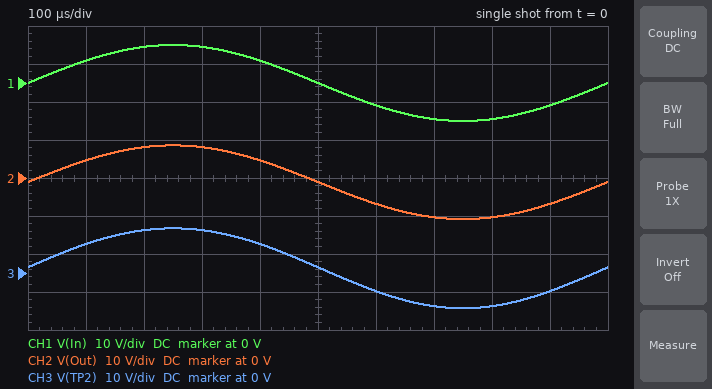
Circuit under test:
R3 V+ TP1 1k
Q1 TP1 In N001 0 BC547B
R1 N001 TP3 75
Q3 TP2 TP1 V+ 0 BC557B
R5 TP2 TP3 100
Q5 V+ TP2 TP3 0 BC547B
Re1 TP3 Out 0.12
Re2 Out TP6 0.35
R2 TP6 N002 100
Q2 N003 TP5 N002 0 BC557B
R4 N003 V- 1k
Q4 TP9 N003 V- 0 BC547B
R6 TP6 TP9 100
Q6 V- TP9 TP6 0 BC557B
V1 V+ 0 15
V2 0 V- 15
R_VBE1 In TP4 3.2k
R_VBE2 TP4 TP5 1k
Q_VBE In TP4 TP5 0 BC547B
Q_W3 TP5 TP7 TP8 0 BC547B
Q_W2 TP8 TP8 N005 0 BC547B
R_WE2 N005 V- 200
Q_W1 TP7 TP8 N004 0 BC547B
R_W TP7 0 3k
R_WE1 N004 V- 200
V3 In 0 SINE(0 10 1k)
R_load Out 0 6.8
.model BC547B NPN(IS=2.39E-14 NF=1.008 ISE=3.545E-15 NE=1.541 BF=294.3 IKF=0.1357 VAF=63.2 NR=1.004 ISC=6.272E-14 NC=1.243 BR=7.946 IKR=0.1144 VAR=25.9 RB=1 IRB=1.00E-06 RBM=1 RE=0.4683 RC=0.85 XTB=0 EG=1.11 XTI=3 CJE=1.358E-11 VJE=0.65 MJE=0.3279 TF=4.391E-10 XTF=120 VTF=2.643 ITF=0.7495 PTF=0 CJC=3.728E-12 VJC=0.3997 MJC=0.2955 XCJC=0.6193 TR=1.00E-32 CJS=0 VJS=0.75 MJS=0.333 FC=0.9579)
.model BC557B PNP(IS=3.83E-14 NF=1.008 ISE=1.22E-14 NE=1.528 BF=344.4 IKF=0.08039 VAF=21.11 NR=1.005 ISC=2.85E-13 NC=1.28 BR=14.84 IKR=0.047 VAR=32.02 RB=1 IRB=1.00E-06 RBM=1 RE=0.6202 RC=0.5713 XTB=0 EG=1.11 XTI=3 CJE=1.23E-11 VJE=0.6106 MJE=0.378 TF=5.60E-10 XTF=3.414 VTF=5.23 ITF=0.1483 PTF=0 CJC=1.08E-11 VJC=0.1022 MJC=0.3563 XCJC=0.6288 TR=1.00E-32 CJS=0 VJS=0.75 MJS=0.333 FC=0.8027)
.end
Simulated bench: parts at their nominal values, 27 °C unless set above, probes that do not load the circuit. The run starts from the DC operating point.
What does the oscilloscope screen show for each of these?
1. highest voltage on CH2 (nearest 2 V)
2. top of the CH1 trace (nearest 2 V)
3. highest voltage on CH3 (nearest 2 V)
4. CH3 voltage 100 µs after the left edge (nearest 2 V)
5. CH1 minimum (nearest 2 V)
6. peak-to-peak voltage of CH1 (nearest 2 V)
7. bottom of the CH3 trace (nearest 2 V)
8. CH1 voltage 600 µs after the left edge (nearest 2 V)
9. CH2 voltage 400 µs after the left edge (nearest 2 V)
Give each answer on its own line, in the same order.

8 V
10 V
12 V
8 V
-10 V
20 V
-10 V
-6 V
4 V
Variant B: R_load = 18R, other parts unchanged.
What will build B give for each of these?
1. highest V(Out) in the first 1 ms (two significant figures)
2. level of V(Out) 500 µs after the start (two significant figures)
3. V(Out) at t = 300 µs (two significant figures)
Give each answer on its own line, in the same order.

8.7 V
-1.1 V
8.3 V
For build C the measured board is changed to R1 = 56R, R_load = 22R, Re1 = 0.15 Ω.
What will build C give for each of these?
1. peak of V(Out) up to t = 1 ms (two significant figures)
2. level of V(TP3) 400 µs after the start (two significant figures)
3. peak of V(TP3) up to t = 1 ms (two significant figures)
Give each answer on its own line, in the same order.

8.7 V
5.1 V
9.2 V
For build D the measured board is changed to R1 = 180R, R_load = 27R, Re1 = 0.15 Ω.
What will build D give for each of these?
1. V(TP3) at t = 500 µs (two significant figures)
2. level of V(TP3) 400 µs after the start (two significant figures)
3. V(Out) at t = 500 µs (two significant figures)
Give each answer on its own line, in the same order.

-870 mV
4.9 V
-1.2 V
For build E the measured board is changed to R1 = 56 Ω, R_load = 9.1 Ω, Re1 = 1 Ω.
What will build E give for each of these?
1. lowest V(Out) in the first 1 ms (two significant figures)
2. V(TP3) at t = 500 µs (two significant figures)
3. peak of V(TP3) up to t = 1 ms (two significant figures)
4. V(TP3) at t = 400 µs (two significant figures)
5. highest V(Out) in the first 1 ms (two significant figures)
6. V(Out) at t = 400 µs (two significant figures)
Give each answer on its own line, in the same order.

-11 V
-670 mV
9.3 V
5.2 V
8.0 V
4.0 V
